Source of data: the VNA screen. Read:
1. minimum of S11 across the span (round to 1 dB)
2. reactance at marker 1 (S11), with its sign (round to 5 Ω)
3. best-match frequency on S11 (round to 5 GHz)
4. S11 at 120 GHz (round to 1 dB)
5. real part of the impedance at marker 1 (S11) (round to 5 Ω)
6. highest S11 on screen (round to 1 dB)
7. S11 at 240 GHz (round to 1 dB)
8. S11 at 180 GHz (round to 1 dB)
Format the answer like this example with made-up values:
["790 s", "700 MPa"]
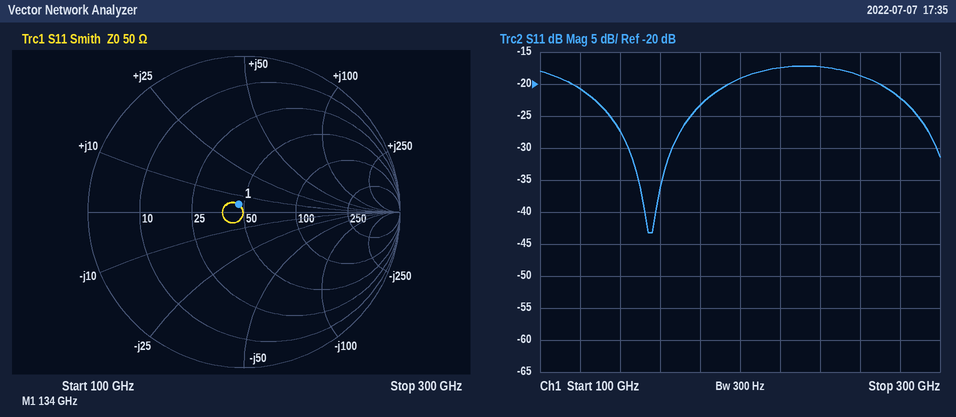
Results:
["-43 dB", "+5 Ω", "155 GHz", "-21 dB", "45 Ω", "-17 dB", "-17 dB", "-23 dB"]
